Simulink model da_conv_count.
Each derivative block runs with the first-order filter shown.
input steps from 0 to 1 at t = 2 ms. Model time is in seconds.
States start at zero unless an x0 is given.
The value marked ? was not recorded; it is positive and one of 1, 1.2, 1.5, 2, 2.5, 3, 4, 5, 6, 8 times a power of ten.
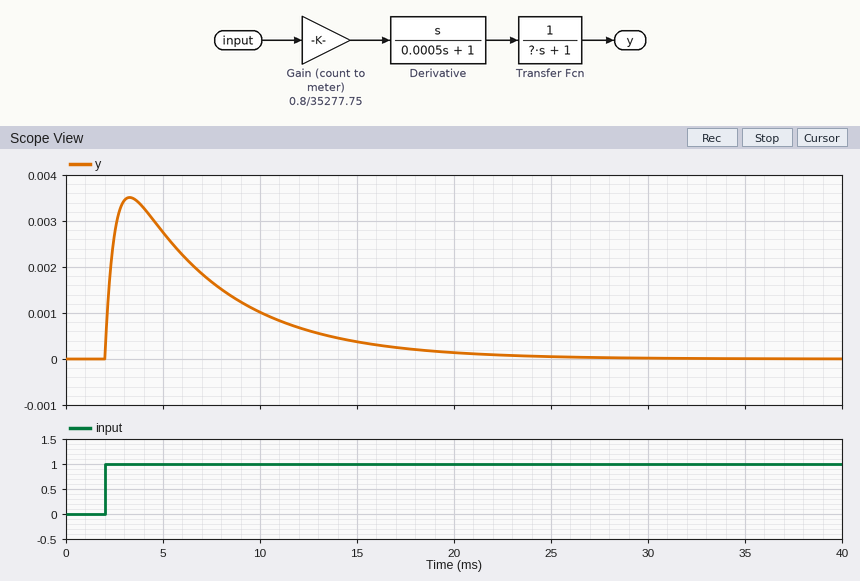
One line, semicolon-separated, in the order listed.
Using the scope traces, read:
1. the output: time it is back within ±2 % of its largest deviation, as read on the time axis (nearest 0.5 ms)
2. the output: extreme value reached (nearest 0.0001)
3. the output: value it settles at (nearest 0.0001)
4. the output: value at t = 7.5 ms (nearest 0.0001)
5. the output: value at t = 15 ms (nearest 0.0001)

23.5 ms; 0.0035; 0.0000; 0.0017; 0.0004
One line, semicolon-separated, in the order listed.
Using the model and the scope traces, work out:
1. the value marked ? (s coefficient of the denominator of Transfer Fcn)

0.005
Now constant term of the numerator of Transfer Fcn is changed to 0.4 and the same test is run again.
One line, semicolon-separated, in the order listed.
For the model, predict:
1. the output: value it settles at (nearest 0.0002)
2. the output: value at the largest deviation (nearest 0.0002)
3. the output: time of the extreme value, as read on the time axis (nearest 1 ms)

0.0000; 0.0014; 3 ms
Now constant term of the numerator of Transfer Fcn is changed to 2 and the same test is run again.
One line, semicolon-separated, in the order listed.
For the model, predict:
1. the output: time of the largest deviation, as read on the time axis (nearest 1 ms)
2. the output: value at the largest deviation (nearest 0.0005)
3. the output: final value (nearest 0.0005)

3 ms; 0.0070; 0.0000
